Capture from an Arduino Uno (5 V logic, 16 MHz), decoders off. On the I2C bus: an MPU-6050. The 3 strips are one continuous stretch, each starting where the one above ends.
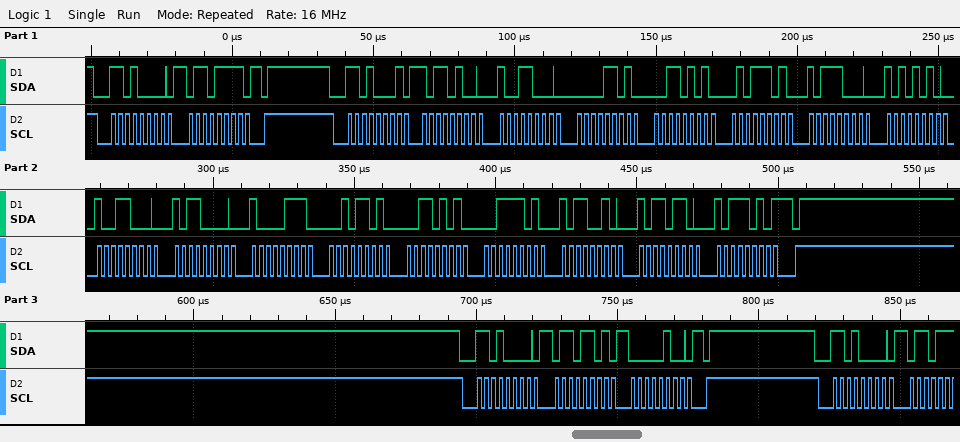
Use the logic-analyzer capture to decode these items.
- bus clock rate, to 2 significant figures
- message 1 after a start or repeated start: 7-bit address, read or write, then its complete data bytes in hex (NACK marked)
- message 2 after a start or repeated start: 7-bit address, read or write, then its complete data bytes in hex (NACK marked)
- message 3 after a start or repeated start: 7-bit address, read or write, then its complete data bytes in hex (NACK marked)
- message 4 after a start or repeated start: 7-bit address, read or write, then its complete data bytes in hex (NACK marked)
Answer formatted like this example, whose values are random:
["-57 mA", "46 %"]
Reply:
["400 kHz", "0x68 write: 6F", "0x68 read: B4 98 0D 35 5D B8 AA 98 B0 87 2D 35 3D B2 B6 BA NACK", "0x68 write: 6D 04", "0x68 write"]
